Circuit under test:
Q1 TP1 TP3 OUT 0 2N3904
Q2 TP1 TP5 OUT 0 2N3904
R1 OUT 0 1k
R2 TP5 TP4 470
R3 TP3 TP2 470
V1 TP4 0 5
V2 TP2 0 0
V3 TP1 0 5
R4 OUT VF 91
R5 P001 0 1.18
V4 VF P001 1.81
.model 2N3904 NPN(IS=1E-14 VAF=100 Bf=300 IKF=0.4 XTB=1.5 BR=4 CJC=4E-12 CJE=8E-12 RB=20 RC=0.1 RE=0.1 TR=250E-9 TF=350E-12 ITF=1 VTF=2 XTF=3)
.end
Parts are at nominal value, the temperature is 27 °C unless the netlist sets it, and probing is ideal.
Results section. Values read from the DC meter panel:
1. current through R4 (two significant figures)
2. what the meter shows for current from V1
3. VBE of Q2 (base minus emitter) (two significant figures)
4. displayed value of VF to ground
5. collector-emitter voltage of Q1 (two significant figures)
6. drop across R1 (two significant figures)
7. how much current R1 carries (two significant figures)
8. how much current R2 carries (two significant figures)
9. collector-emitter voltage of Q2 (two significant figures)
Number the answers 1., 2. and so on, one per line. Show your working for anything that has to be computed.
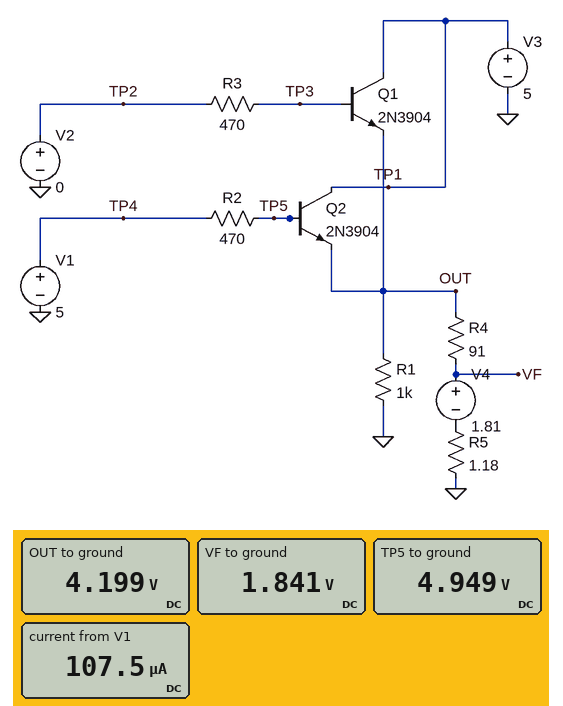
1. (4.199 V - 1.841 V) / 91 Ω = 26 mA
2. 107.5 µA
3. 4.949 V - 4.199 V = 750 mV
4. 1.841 V
5. 5 V - 4.199 V = 800 mV
6. 4.199 V = 4.2 V
7. (4.199 V) / 1 kΩ = 4.2 mA
8. (5 V - 4.949 V) / 470 Ω = 110 µA
9. 5 V - 4.199 V = 800 mV
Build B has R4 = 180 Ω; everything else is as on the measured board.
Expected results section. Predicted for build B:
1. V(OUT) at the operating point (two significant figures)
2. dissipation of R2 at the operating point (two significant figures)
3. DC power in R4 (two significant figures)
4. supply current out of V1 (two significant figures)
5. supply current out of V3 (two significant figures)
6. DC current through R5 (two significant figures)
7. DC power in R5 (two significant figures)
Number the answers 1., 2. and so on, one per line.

1. 4.2 V
2. 1.8 µW
3. 32 mW
4. 61 µA
5. 18 mA
6. 13 mA
7. 210 µW
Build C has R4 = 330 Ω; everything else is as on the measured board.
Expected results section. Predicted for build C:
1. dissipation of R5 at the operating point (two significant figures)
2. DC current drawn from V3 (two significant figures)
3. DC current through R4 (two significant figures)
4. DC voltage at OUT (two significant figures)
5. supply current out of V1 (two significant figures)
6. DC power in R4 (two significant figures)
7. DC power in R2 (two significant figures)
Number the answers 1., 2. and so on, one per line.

1. 65 µW
2. 12 mA
3. 7.4 mA
4. 4.3 V
5. 40 µA
6. 18 mW
7. 750 nW
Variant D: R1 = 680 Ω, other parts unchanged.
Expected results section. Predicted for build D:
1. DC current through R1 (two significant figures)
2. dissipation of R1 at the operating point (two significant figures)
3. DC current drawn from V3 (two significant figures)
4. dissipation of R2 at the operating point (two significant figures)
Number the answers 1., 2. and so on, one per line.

1. 6.2 mA
2. 26 mW
3. 32 mA
4. 6.2 µW
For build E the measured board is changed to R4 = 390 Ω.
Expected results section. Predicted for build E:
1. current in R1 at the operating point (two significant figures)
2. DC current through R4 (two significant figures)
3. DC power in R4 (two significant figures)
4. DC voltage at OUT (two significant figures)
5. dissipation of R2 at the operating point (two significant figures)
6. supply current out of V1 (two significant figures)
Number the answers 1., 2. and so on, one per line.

1. 4.3 mA
2. 6.3 mA
3. 15 mW
4. 4.3 V
5. 610 nW
6. 36 µA
